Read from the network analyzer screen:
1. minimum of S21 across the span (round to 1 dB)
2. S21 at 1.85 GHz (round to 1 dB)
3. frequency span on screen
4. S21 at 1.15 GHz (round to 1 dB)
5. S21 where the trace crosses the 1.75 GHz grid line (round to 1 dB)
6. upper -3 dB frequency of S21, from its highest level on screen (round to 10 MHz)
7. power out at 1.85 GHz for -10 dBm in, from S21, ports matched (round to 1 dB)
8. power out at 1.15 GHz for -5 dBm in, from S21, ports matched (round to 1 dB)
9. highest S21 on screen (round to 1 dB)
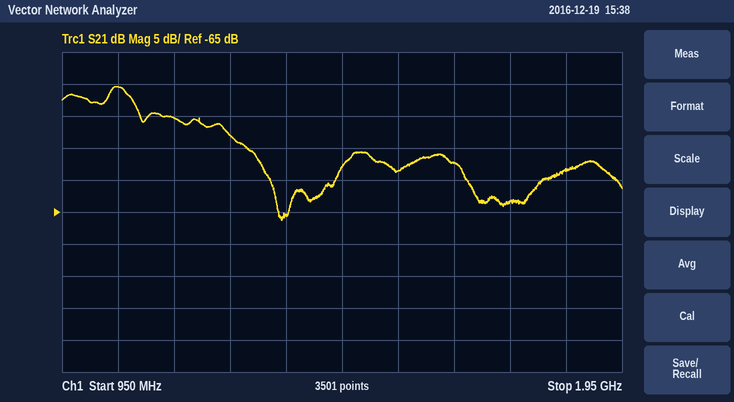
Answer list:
-66 dB
-58 dB
1 GHz
-50 dB
-63 dB
1.08 GHz
-68 dBm
-55 dBm
-45 dB
